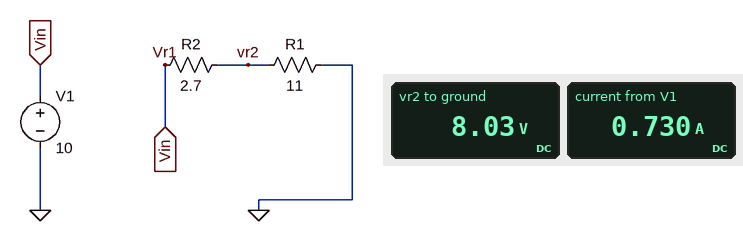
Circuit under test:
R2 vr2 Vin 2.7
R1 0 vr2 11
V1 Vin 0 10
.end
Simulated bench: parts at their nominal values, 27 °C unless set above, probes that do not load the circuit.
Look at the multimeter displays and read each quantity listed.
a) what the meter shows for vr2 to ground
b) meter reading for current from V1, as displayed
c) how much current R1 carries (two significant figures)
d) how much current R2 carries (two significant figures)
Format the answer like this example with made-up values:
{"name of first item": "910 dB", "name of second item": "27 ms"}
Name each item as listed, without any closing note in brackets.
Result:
{"what the meter shows for vr2 to ground": "8.03 V", "meter reading for current from V1, as displayed": "0.730 A", "how much current R1 carries": "730 mA", "how much current R2 carries": "730 mA"}
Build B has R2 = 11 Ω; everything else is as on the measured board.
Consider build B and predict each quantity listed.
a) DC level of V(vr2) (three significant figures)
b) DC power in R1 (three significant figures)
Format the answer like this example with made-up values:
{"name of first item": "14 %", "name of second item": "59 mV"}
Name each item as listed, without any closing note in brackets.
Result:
{"DC level of V(vr2)": "5.00 V", "DC power in R1": "2.27 W"}
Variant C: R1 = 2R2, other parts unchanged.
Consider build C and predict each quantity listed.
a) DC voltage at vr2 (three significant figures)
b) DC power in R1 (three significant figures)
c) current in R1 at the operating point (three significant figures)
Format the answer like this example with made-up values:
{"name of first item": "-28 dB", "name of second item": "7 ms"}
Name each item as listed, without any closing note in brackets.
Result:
{"DC voltage at vr2": "4.49 V", "DC power in R1": "9.16 W", "current in R1 at the operating point": "2.04 A"}
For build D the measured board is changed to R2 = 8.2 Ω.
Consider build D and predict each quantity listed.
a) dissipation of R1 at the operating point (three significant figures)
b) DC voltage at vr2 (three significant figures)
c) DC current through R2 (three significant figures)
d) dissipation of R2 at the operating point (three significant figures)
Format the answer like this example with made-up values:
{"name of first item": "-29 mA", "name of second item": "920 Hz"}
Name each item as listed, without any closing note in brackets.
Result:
{"dissipation of R1 at the operating point": "2.98 W", "DC voltage at vr2": "5.73 V", "DC current through R2": "521 mA", "dissipation of R2 at the operating point": "2.22 W"}
